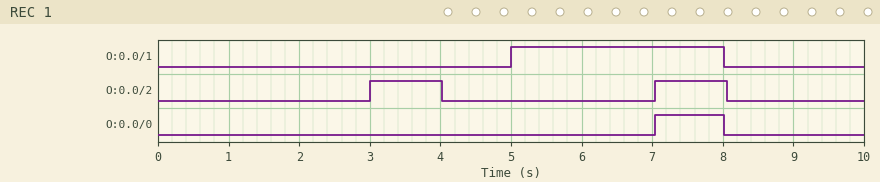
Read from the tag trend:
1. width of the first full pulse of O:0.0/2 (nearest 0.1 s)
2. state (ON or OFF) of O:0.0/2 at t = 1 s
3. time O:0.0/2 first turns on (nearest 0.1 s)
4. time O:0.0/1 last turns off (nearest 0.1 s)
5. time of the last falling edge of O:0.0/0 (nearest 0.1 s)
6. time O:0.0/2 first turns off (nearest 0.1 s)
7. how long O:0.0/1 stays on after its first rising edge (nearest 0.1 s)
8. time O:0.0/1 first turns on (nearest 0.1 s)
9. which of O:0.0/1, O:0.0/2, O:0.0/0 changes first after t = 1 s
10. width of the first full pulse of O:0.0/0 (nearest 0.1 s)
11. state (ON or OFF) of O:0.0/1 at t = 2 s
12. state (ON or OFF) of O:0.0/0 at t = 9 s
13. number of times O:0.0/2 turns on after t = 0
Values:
1.0 s
OFF
3.0 s
8.0 s
8.0 s
4.0 s
3.0 s
5.0 s
O:0.0/2
1.0 s
OFF
OFF
2
